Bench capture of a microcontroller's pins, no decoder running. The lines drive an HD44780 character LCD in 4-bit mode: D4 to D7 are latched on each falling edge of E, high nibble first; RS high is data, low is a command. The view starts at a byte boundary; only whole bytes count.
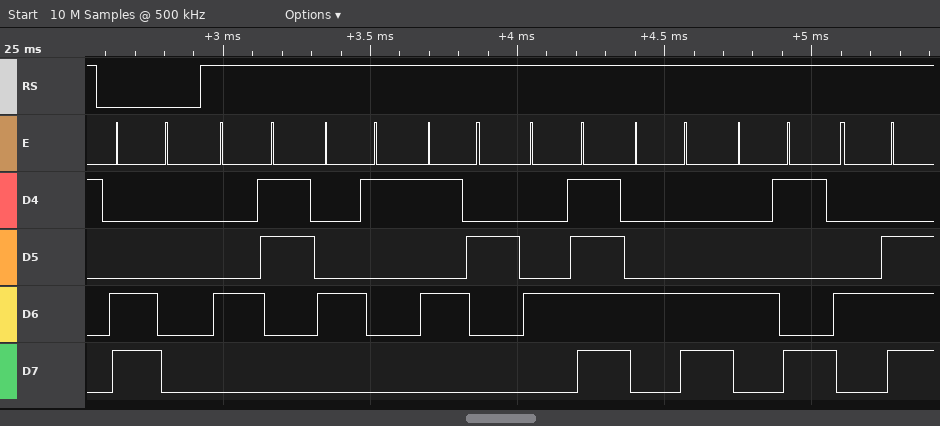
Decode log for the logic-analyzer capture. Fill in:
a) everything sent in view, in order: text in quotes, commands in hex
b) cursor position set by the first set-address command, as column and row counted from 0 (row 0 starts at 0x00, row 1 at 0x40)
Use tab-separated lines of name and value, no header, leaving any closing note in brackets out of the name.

everything sent in view, in order: text in quotes, commands in hex	0xC0 "CAROLIN"
cursor position set by the first set-address command, as column and row counted from 0	column 0, row 1
